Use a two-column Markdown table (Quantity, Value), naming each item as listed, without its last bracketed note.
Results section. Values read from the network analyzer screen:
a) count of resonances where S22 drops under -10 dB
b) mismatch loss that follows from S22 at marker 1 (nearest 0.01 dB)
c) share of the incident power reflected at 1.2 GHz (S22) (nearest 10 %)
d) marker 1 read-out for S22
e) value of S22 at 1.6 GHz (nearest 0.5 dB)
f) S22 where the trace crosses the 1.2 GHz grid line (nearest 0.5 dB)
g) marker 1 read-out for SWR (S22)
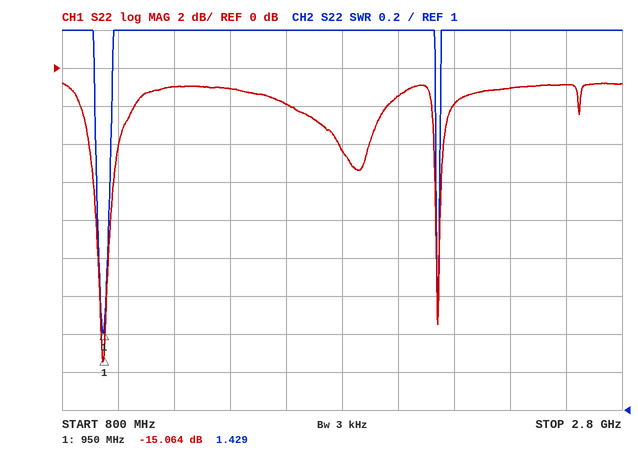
| Quantity | Value |
|---|---|
| count of resonances where S22 drops under -10 dB | 2 |
| mismatch loss that follows from S22 at marker 1 | 0.14 dB |
| share of the incident power reflected at 1.2 GHz (S22) | 80 % |
| marker 1 read-out for S22 | -15.064 dB |
| value of S22 at 1.6 GHz | -2.0 dB |
| S22 where the trace crosses the 1.2 GHz grid line | -1.0 dB |
| marker 1 read-out for SWR | 1.429 |
